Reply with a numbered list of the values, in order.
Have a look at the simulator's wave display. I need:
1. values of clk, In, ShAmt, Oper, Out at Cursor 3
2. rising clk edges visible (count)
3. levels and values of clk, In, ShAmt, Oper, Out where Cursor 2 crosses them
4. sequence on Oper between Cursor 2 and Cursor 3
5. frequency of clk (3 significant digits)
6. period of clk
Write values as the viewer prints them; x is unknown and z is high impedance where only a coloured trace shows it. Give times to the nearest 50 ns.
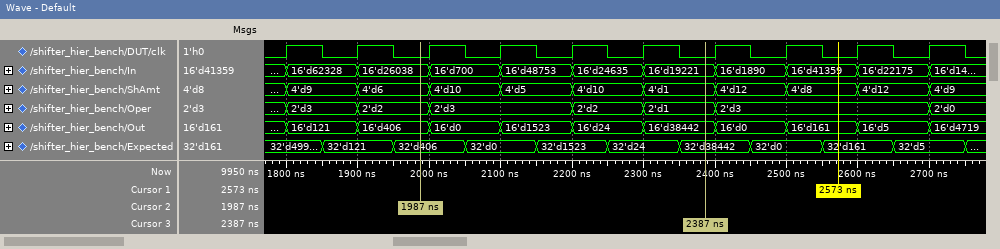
1. clk=0, In=16'd19221, ShAmt=4'd1, Oper=2'd1, Out=16'd38442
2. 10
3. clk=0, In=16'd26038, ShAmt=4'd6, Oper=2'd2, Out=16'd406
4. 2'd2, 2'd3, 2'd2, 2'd1
5. 10.0 MHz
6. 100 ns
